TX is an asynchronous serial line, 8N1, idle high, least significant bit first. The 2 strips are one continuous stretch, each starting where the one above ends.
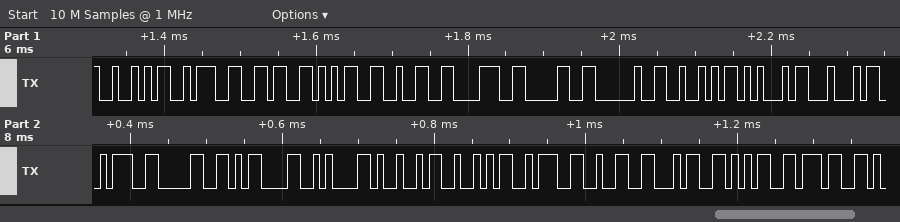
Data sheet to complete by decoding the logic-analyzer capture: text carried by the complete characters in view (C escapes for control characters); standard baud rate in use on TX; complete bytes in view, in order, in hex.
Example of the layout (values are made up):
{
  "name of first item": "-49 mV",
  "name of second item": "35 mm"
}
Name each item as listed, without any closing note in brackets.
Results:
{
  "text carried by the complete characters in view": "\"R:65280 RED:0\\r\\nIR:2457\"",
  "standard baud rate in use on TX": "115200 baud",
  "complete bytes in view, in order, in hex": "52 3A 36 35 32 38 30 20 52 45 44 3A 30 0D 0A 49 52 3A 32 34 35 37"
}
